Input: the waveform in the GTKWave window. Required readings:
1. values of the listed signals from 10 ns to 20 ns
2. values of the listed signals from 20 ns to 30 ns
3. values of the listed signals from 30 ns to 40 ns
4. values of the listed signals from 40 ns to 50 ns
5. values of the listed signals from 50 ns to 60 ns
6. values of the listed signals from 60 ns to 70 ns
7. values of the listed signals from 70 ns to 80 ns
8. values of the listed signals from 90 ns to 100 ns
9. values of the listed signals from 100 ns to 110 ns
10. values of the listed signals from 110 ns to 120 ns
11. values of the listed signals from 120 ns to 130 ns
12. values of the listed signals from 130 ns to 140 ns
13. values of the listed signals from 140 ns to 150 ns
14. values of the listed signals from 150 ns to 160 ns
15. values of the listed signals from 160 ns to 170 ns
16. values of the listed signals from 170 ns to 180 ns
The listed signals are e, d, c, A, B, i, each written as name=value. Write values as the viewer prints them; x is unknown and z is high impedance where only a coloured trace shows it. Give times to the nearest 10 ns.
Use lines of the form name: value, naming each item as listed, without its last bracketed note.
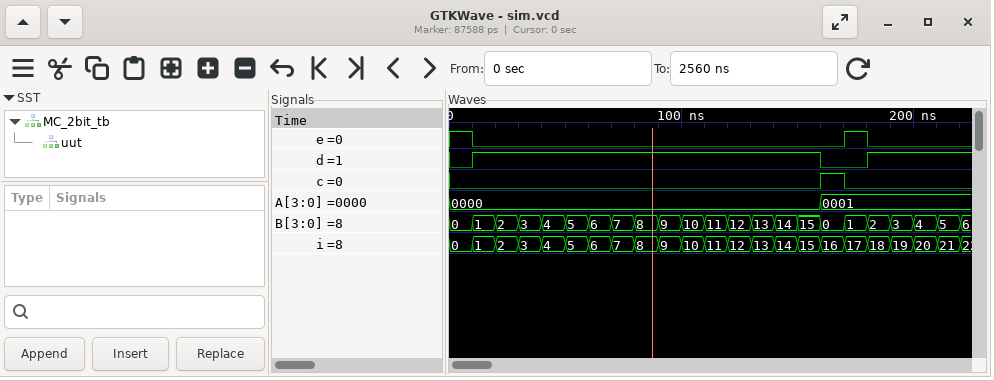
values of the listed signals from 10 ns to 20 ns: e=0, d=1, c=0, A=0000, B=1, i=1
values of the listed signals from 20 ns to 30 ns: e=0, d=1, c=0, A=0000, B=2, i=2
values of the listed signals from 30 ns to 40 ns: e=0, d=1, c=0, A=0000, B=3, i=3
values of the listed signals from 40 ns to 50 ns: e=0, d=1, c=0, A=0000, B=4, i=4
values of the listed signals from 50 ns to 60 ns: e=0, d=1, c=0, A=0000, B=5, i=5
values of the listed signals from 60 ns to 70 ns: e=0, d=1, c=0, A=0000, B=6, i=6
values of the listed signals from 70 ns to 80 ns: e=0, d=1, c=0, A=0000, B=7, i=7
values of the listed signals from 90 ns to 100 ns: e=0, d=1, c=0, A=0000, B=9, i=9
values of the listed signals from 100 ns to 110 ns: e=0, d=1, c=0, A=0000, B=10, i=10
values of the listed signals from 110 ns to 120 ns: e=0, d=1, c=0, A=0000, B=11, i=11
values of the listed signals from 120 ns to 130 ns: e=0, d=1, c=0, A=0000, B=12, i=12
values of the listed signals from 130 ns to 140 ns: e=0, d=1, c=0, A=0000, B=13, i=13
values of the listed signals from 140 ns to 150 ns: e=0, d=1, c=0, A=0000, B=14, i=14
values of the listed signals from 150 ns to 160 ns: e=0, d=1, c=0, A=0000, B=15, i=15
values of the listed signals from 160 ns to 170 ns: e=0, d=0, c=1, A=0001, B=0, i=16
values of the listed signals from 170 ns to 180 ns: e=1, d=0, c=0, A=0001, B=1, i=17
